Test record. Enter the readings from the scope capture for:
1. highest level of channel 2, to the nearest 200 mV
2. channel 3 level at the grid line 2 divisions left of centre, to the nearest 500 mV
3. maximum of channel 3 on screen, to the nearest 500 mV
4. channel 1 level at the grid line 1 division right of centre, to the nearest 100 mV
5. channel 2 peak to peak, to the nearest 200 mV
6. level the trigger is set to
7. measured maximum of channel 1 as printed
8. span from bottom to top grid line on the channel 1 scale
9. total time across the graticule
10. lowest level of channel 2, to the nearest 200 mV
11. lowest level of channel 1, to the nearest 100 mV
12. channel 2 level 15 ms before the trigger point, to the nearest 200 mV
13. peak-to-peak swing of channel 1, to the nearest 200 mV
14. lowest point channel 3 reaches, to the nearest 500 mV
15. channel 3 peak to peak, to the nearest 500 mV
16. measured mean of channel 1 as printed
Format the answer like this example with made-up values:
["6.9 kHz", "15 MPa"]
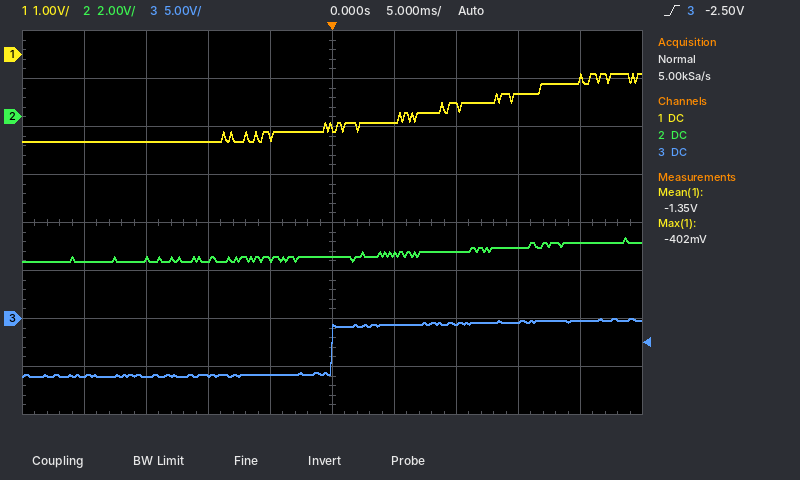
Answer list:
["-5.0 V", "-6.0 V", "0.0 V", "-1.4 V", "1.0 V", "-2.50 V", "-402 mV", "8 V", "50 ms", "-6.0 V", "-1.8 V", "-6.0 V", "1.4 V", "-6.0 V", "6.0 V", "-1.35 V"]
